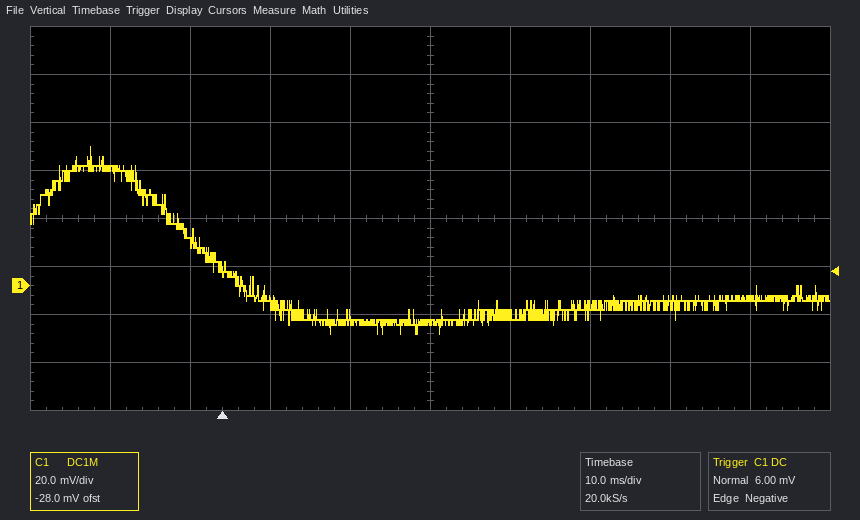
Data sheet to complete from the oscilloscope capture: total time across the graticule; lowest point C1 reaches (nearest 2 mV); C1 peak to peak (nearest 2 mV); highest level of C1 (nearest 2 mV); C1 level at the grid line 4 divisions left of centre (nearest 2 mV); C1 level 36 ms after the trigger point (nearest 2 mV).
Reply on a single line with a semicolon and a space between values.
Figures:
100 ms; -20 mV; 78 mV; 58 mV; 48 mV; -12 mV
